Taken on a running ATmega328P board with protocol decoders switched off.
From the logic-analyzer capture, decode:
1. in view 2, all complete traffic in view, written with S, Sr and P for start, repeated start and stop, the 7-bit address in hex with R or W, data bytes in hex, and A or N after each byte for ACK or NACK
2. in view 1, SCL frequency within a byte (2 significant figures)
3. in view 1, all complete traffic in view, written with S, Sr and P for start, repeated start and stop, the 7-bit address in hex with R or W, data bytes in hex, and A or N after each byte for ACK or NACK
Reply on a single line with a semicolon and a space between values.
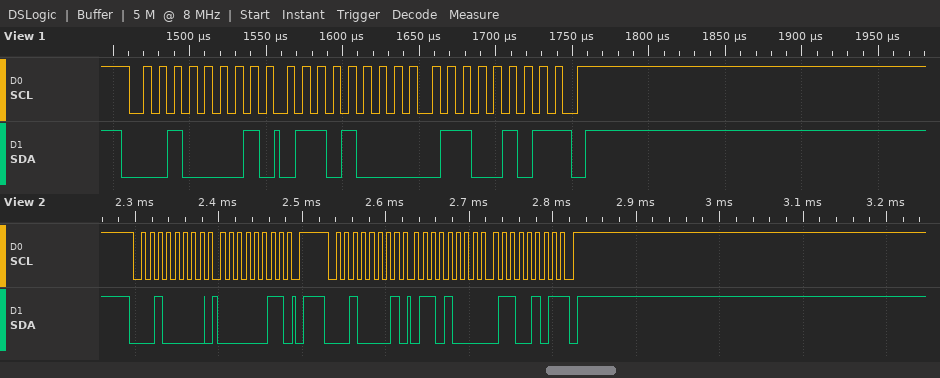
S 10W A 03 A P S 10R A 68 A 65 N P; 100 kHz; S 10R A 68 A 65 N P
